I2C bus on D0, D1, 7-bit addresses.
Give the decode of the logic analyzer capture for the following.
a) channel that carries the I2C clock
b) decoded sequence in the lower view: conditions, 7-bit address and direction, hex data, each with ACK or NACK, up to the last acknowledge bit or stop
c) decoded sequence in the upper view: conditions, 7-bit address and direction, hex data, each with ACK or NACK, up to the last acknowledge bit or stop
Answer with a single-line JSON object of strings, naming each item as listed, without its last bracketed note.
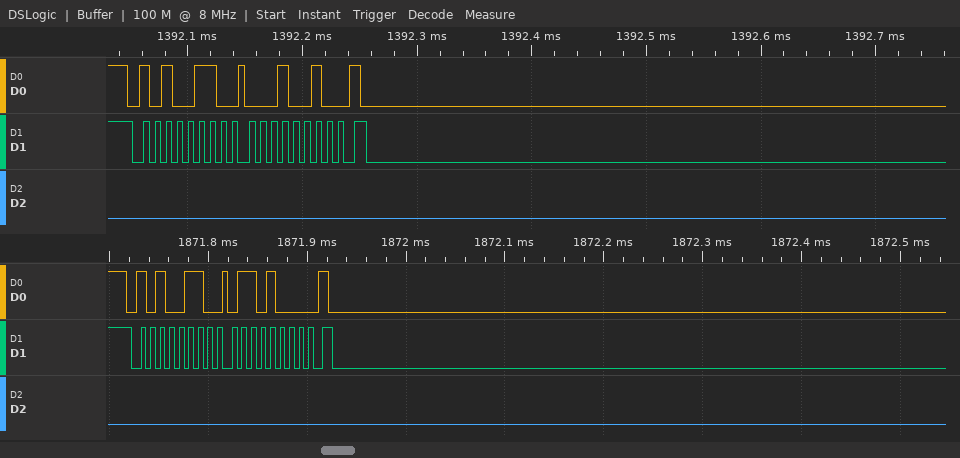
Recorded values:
{"channel that carries the I2C clock": "D1", "decoded sequence in the lower view: conditions, 7-bit address and direction, hex data, each with ACK or NACK, up to the last acknowledge bit or stop": "start, address 53 write ACK, 68 ACK", "decoded sequence in the upper view: conditions, 7-bit address and direction, hex data, each with ACK or NACK, up to the last acknowledge bit or stop": "start, address 53 write ACK, 12 ACK"}
